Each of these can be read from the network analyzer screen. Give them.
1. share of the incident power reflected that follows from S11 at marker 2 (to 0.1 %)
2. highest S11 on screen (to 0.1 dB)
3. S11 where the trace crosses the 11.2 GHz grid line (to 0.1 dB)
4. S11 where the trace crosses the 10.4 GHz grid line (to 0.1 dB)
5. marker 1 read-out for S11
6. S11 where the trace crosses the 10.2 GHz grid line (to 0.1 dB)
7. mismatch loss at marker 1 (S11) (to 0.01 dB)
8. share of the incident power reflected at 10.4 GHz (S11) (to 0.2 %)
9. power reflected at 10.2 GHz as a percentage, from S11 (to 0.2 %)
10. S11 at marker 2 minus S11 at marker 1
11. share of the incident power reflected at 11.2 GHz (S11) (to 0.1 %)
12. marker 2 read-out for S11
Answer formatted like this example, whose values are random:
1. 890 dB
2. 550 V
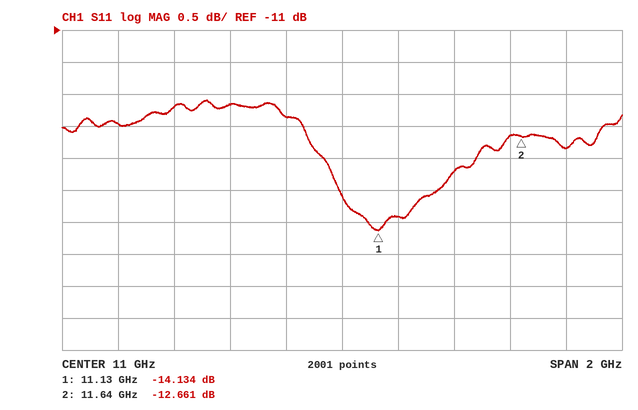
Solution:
1. 5.4 %
2. -12.1 dB
3. -13.9 dB
4. -12.2 dB
5. -14.134 dB
6. -12.5 dB
7. 0.17 dB
8. 6.0 %
9. 5.6 %
10. 1.473 dB
11. 4.1 %
12. -12.661 dB
